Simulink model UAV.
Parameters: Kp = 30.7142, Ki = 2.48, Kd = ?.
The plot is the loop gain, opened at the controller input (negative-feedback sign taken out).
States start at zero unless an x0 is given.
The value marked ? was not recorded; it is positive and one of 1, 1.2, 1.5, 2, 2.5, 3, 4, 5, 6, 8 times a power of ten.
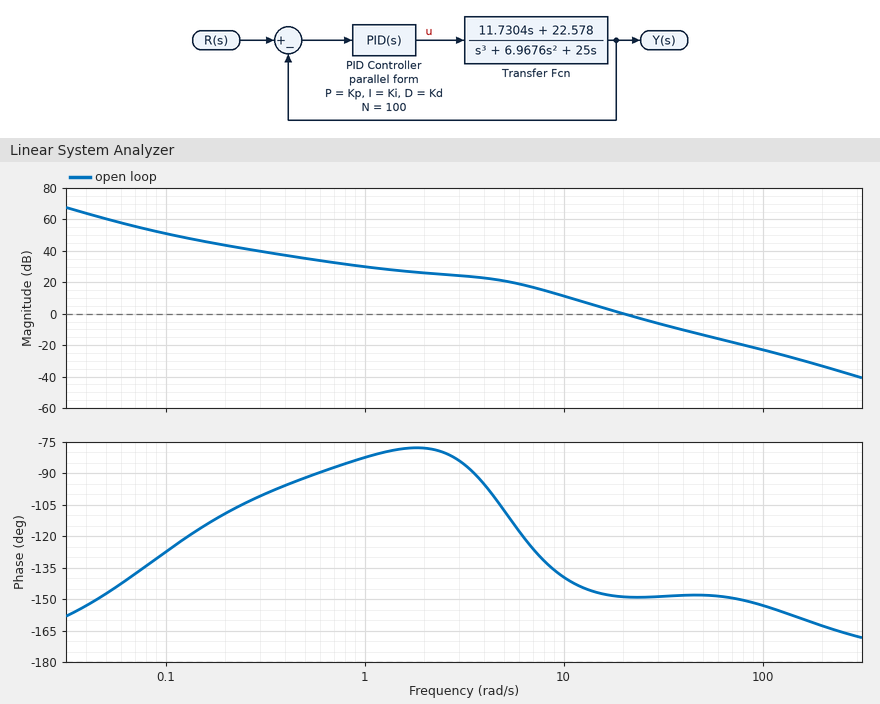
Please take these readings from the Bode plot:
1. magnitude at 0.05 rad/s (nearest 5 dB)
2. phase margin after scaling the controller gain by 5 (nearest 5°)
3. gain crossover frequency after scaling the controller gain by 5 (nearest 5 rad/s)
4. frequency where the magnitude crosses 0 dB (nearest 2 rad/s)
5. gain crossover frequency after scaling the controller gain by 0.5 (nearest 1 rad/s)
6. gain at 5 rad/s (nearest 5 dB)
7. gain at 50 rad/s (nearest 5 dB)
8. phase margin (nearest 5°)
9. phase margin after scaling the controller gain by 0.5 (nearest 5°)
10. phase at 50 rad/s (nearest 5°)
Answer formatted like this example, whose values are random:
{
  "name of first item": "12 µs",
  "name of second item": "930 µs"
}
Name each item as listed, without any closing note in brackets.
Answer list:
{
  "magnitude at 0.05 rad/s": "60 dB",
  "phase margin after scaling the controller gain by 5": "30°",
  "gain crossover frequency after scaling the controller gain by 5": "50 rad/s",
  "frequency where the magnitude crosses 0 dB": "20 rad/s",
  "gain crossover frequency after scaling the controller gain by 0.5": "14 rad/s",
  "gain at 5 rad/s": "20 dB",
  "gain at 50 rad/s": "-15 dB",
  "phase margin": "30°",
  "phase margin after scaling the controller gain by 0.5": "35°",
  "phase at 50 rad/s": "-150°"
}
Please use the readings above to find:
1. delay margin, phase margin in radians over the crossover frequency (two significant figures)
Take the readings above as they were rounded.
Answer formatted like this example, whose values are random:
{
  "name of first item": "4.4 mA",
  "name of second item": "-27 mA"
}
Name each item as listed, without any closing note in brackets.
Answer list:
{
  "delay margin, phase margin in radians over the crossover frequency": "0.026 s"
}
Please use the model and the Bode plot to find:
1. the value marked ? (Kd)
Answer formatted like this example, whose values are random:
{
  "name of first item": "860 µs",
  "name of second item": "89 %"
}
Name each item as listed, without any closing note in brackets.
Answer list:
{
  "the value marked ?": "0.5"
}
